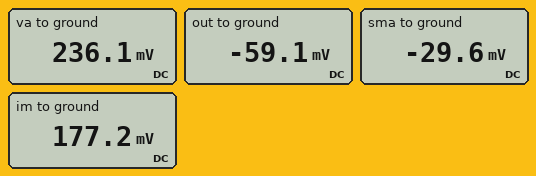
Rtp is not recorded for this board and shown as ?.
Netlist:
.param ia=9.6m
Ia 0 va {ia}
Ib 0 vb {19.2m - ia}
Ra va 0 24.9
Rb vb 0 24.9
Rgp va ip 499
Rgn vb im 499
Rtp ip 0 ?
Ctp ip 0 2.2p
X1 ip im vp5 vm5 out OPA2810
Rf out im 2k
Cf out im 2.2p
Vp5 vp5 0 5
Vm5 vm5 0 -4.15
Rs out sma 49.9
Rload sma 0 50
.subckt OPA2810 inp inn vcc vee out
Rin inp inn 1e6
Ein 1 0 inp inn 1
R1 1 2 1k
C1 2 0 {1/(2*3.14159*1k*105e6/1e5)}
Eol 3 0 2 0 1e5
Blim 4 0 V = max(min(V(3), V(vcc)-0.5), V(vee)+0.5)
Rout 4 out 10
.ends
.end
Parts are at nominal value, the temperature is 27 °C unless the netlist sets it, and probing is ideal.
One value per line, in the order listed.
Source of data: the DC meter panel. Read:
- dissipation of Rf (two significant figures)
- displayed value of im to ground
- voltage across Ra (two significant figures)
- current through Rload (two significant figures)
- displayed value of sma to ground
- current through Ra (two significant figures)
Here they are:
28 µW
177.2 mV
240 mV
590 µA
-29.6 mV
9.5 mA
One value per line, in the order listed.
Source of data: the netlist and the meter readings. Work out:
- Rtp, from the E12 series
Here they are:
1.5 kΩ
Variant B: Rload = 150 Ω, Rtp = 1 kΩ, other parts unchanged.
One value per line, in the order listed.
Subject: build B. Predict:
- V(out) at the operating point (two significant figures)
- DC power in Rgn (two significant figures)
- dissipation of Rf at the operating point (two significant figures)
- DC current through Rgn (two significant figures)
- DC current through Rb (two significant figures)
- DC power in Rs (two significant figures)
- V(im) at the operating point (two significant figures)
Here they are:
-160 mV
12 µW
49 µW
160 µA
9.4 mA
31 µW
160 mV
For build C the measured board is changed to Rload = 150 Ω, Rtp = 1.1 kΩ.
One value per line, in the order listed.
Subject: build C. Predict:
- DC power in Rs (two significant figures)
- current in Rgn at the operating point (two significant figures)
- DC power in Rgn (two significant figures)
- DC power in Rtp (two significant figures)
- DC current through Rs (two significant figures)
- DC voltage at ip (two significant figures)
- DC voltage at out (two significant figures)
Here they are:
22 µW
150 µA
11 µW
24 µW
660 µA
160 mV
-130 mV
